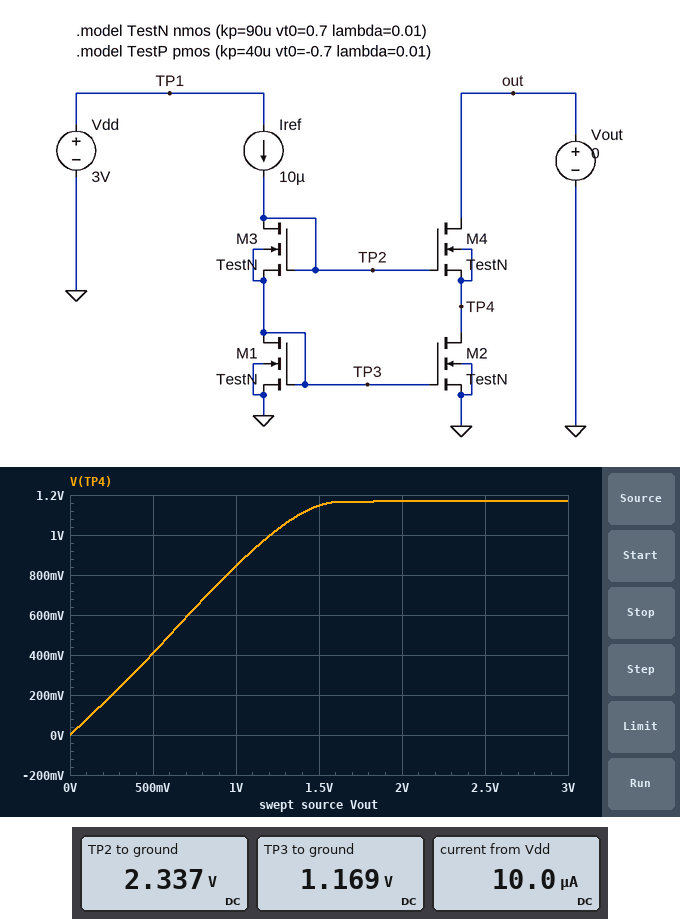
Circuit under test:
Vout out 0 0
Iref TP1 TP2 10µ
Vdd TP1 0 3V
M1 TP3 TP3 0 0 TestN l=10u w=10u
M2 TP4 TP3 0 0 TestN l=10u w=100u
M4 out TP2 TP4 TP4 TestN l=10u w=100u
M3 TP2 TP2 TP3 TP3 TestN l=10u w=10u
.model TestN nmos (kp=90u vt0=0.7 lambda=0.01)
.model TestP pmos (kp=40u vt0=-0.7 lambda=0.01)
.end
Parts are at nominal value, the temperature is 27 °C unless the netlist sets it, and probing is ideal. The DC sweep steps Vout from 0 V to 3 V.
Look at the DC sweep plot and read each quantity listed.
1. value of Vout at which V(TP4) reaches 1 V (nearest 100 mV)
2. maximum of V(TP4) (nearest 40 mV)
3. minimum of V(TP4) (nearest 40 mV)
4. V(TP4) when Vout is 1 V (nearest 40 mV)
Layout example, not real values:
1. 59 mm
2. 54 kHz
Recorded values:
1. 1.2 V
2. 1.16 V
3. 0 V
4. 840 mV
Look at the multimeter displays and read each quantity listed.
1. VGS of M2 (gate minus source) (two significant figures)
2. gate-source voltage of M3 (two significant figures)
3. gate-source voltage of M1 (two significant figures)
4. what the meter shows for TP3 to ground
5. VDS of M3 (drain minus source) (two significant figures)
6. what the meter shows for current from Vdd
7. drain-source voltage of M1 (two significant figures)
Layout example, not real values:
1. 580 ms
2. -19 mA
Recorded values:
1. 1.2 V
2. 1.2 V
3. 1.2 V
4. 1.169 V
5. 1.2 V
6. 10.0 µA
7. 1.2 V
